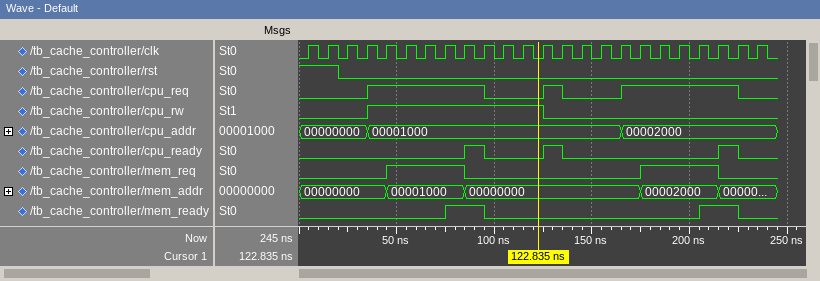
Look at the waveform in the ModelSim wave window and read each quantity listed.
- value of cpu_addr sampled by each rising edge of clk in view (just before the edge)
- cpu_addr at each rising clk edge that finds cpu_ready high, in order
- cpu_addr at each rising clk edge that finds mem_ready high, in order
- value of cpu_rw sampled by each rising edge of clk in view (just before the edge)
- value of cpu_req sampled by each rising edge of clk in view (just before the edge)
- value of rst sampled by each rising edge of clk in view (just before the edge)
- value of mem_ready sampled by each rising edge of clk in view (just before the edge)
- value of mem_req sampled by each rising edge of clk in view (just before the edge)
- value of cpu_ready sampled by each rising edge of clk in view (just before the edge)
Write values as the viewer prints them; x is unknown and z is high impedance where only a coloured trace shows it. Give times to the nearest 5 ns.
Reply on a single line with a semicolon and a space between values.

00000000, 00000000, 00000000, 00000000, 00001000, 00001000, 00001000, 00001000, 00001000, 00001000, 00001000, 00001000, 00001000, 00001000, 00001000, 00001000, 00001000, 00002000, 00002000, 00002000, 00002000, 00002000, 00002000, 00002000; 00001000, 00001000, 00002000; 00001000, 00001000, 00002000, 00002000; 0 0 0 0 1 1 1 1 1 1 1 1 1 0 0 0 0 0 0 0 0 0 0 0; 0 0 0 0 1 1 1 1 1 1 0 0 0 1 0 0 0 1 1 1 1 1 1 0; 1 1 0 0 0 0 0 0 0 0 0 0 0 0 0 0 0 0 0 0 0 0 0 0; 0 0 0 0 0 0 0 0 1 1 0 0 0 0 0 0 0 0 0 0 0 1 1 0; 0 0 0 0 0 1 1 1 1 0 0 0 0 0 0 0 0 0 1 1 1 1 0 0; 0 0 0 0 0 0 0 0 0 1 0 0 0 1 0 0 0 0 0 0 0 0 1 0
